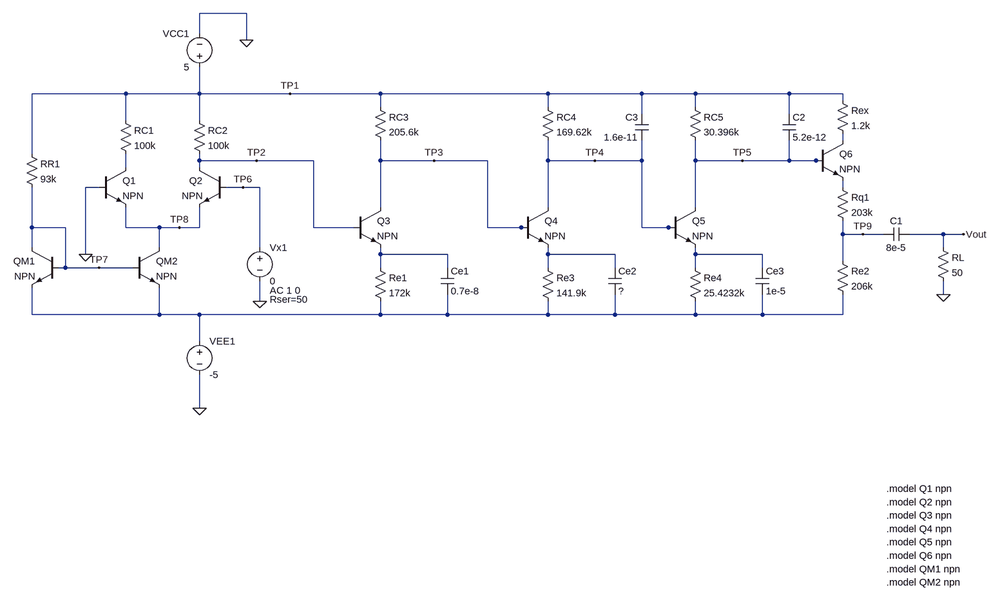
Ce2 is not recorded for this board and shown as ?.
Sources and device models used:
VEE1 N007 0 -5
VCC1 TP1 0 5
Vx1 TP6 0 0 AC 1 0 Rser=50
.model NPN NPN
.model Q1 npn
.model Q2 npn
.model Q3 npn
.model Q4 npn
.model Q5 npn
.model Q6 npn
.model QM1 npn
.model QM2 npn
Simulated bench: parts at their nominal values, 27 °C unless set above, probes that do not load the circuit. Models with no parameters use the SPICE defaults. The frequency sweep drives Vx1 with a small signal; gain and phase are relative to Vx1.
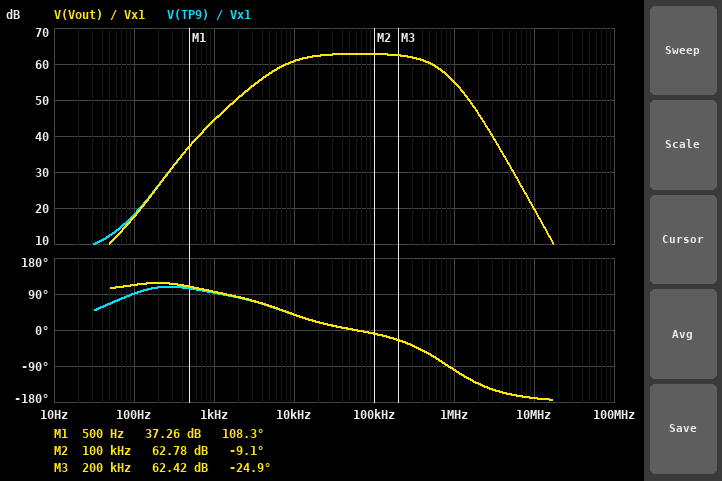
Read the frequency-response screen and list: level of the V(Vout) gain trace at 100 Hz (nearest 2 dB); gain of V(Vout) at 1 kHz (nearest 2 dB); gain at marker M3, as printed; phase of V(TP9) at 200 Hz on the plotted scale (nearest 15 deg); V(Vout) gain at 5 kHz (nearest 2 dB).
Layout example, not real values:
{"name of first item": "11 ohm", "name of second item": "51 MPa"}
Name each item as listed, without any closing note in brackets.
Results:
{"level of the V(Vout) gain trace at 100 Hz": "18 dB", "gain of V(Vout) at 1 kHz": "44 dB", "gain at marker M3, as printed": "62.42 dB", "phase of V(TP9) at 200 Hz on the plotted scale": "105 deg", "V(Vout) gain at 5 kHz": "58 dB"}
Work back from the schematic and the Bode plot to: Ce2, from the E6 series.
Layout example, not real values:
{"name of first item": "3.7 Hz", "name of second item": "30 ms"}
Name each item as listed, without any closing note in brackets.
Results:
{"Ce2, from the E6 series": "150 nF"}
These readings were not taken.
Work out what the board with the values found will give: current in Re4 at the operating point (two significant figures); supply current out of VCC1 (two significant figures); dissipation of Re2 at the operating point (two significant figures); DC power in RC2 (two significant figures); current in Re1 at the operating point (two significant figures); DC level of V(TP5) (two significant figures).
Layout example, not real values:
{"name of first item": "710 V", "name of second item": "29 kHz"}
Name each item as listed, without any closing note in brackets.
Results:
{"current in Re4 at the operating point": "170 µA", "supply current out of VCC1": "430 µA", "dissipation of Re2 at the operating point": "23 µW", "DC power in RC2": "240 µW", "current in Re1 at the operating point": "26 µA", "DC level of V(TP5)": "-50 mV"}
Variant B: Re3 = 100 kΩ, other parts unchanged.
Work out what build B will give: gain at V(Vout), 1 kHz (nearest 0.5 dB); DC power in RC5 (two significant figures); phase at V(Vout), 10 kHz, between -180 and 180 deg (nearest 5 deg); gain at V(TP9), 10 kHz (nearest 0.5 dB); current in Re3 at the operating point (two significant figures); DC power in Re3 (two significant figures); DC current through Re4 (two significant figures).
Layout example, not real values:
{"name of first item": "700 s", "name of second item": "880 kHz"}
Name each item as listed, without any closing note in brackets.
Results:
{"gain at V(Vout), 1 kHz": "-9.5 dB", "DC power in RC5": "450 µW", "phase at V(Vout), 10 kHz, between -180 and 180 deg": "50 deg", "gain at V(TP9), 10 kHz": "6.0 dB", "current in Re3 at the operating point": "38 µA", "DC power in Re3": "140 µW", "DC current through Re4": "120 µA"}
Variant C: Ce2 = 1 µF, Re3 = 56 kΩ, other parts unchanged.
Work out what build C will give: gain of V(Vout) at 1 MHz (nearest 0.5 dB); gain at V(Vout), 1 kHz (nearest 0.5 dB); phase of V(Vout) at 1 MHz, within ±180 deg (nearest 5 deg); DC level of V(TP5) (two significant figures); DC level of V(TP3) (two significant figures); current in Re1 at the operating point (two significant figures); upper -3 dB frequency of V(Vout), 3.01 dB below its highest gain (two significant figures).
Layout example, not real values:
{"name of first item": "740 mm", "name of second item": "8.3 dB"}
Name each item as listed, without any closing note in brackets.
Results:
{"gain of V(Vout) at 1 MHz": "-35.5 dB", "gain at V(Vout), 1 kHz": "-33.5 dB", "phase of V(Vout) at 1 MHz, within ±180 deg": "-45 deg", "DC level of V(TP5)": "2.1 V", "DC level of V(TP3)": "-1.2 V", "current in Re1 at the operating point": "22 µA", "upper -3 dB frequency of V(Vout), 3.01 dB below its highest gain": "100 Hz"}
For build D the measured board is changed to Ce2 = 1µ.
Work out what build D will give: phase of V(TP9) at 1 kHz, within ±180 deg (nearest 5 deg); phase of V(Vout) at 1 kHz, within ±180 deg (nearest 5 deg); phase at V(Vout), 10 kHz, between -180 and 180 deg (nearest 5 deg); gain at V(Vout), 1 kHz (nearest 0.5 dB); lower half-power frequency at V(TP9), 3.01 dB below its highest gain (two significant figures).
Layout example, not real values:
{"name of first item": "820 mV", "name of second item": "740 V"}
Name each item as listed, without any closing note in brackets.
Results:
{"phase of V(TP9) at 1 kHz, within ±180 deg": "75 deg", "phase of V(Vout) at 1 kHz, within ±180 deg": "80 deg", "phase at V(Vout), 10 kHz, between -180 and 180 deg": "35 deg", "gain at V(Vout), 1 kHz": "45.0 dB", "lower half-power frequency at V(TP9), 3.01 dB below its highest gain": "7.6 kHz"}
